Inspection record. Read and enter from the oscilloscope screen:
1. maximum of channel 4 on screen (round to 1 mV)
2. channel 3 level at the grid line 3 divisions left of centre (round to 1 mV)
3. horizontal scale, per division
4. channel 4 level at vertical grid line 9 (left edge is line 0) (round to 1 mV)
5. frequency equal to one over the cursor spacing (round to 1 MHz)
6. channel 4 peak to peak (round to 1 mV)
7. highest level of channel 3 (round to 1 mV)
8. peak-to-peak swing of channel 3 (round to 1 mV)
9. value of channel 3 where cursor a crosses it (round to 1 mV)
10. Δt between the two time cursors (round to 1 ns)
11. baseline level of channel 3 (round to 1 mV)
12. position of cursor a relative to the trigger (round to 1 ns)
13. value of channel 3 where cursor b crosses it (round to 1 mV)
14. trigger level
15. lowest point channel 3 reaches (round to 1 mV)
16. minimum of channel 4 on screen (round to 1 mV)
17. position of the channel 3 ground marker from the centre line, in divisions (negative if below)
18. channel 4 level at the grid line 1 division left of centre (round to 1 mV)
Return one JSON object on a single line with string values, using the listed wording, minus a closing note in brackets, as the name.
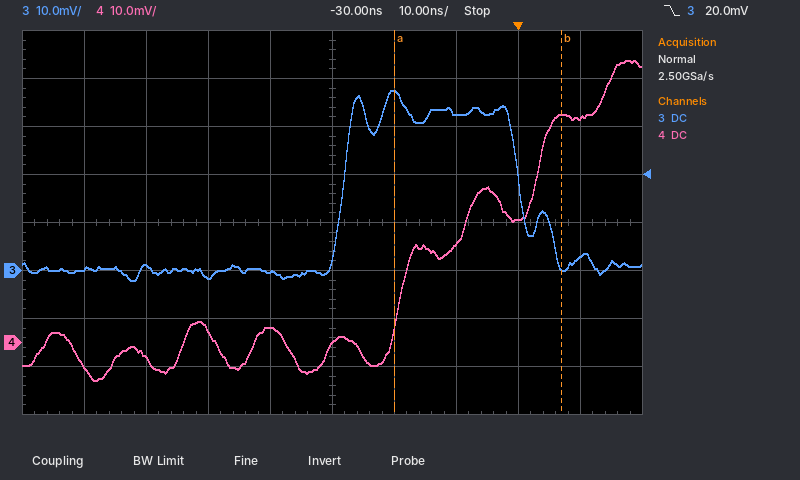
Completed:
{"maximum of channel 4 on screen": "59 mV", "channel 3 level at the grid line 3 divisions left of centre": "1 mV", "horizontal scale, per division": "10 ns", "channel 4 level at vertical grid line 9 (left edge is line 0)": "47 mV", "frequency equal to one over the cursor spacing": "37 MHz", "channel 4 peak to peak": "67 mV", "highest level of channel 3": "38 mV", "peak-to-peak swing of channel 3": "40 mV", "value of channel 3 where cursor a crosses it": "37 mV", "Δt between the two time cursors": "27 ns", "baseline level of channel 3": "0 mV", "position of cursor a relative to the trigger": "-20 ns", "value of channel 3 where cursor b crosses it": "1 mV", "trigger level": "20.0 mV", "lowest point channel 3 reaches": "-2 mV", "minimum of channel 4 on screen": "-8 mV", "position of the channel 3 ground marker from the centre line, in divisions": "-1.0 div", "channel 4 level at the grid line 1 division left of centre": "3 mV"}
